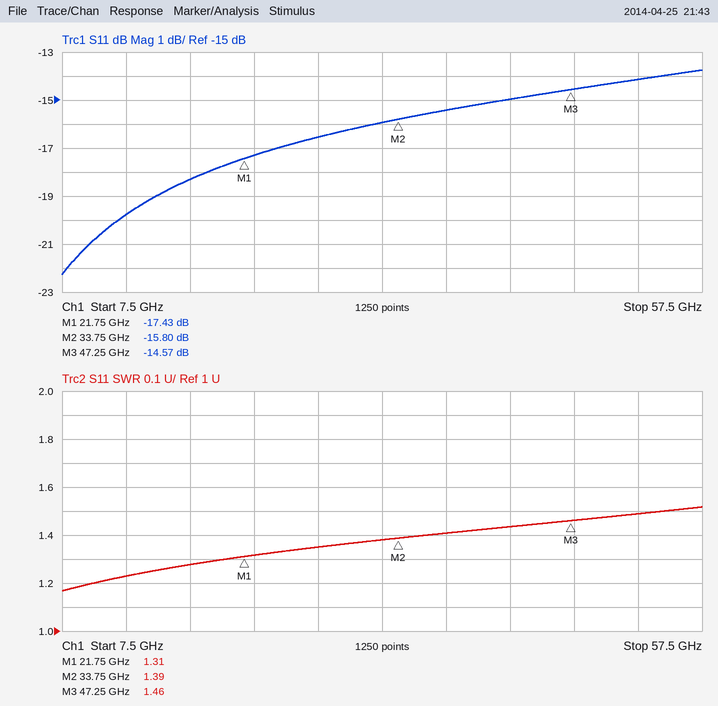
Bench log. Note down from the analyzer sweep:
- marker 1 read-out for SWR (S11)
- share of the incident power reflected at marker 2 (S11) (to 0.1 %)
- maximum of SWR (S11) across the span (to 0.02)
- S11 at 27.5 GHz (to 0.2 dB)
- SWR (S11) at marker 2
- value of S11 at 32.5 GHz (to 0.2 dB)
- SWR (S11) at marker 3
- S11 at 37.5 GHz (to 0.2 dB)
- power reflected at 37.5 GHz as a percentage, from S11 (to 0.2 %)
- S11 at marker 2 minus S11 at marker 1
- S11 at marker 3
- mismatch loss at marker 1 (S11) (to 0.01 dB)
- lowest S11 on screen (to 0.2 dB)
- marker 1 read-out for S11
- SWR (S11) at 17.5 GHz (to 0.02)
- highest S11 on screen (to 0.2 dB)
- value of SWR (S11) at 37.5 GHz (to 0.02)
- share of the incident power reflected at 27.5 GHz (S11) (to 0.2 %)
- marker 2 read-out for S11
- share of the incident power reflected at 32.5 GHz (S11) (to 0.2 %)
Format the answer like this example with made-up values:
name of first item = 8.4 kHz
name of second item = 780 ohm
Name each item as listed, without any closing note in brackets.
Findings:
marker 1 read-out for SWR = 1.31
share of the incident power reflected at marker 2 (S11) = 2.6 %
maximum of SWR (S11) across the span = 1.52
S11 at 27.5 GHz = -16.6 dB
SWR (S11) at marker 2 = 1.39
value of S11 at 32.5 GHz = -16.0 dB
SWR (S11) at marker 3 = 1.46
S11 at 37.5 GHz = -15.4 dB
power reflected at 37.5 GHz as a percentage, from S11 = 2.8 %
S11 at marker 2 minus S11 at marker 1 = 1.63 dB
S11 at marker 3 = -14.57 dB
mismatch loss at marker 1 (S11) = 0.08 dB
lowest S11 on screen = -22.2 dB
marker 1 read-out for S11 = -17.43 dB
SWR (S11) at 17.5 GHz = 1.28
highest S11 on screen = -13.8 dB
value of SWR (S11) at 37.5 GHz = 1.40
share of the incident power reflected at 27.5 GHz (S11) = 2.2 %
marker 2 read-out for S11 = -15.80 dB
share of the incident power reflected at 32.5 GHz (S11) = 2.6 %
